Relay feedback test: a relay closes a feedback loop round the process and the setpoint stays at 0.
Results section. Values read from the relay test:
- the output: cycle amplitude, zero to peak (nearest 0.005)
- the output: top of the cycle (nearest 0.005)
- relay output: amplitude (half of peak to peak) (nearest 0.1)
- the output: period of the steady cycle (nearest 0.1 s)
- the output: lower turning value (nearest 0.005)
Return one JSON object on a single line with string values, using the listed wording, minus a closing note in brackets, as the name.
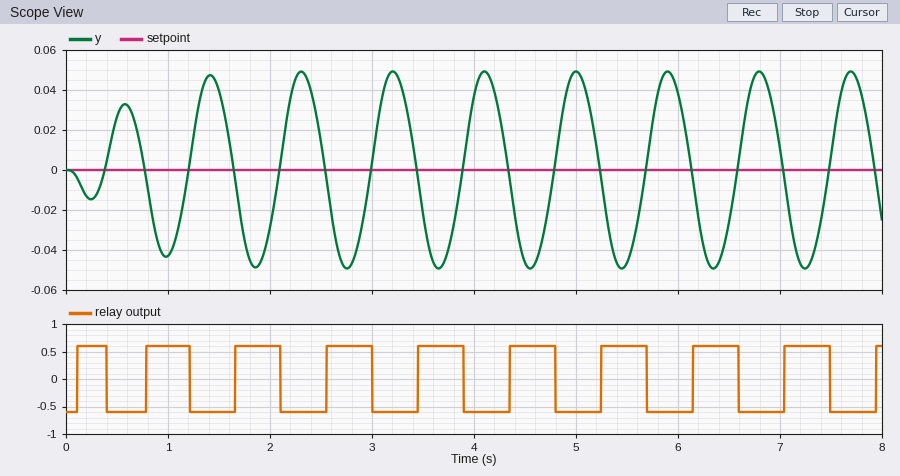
{"the output: cycle amplitude, zero to peak": "0.050", "the output: top of the cycle": "0.050", "relay output: amplitude (half of peak to peak)": "0.6", "the output: period of the steady cycle": "0.9 s", "the output: lower turning value": "-0.050"}
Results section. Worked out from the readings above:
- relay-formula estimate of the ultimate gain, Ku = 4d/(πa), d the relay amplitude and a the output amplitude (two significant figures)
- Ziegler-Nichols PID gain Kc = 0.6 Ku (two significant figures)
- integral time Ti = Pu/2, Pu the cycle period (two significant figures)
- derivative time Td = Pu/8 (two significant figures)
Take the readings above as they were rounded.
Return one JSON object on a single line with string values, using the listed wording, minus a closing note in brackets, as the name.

{"relay-formula estimate of the ultimate gain, Ku = 4d/(πa), d the relay amplitude and a the output amplitude": "15", "Ziegler-Nichols PID gain Kc = 0.6 Ku": "9.0", "integral time Ti = Pu/2, Pu the cycle period": "0.45 s", "derivative time Td = Pu/8": "0.11 s"}
